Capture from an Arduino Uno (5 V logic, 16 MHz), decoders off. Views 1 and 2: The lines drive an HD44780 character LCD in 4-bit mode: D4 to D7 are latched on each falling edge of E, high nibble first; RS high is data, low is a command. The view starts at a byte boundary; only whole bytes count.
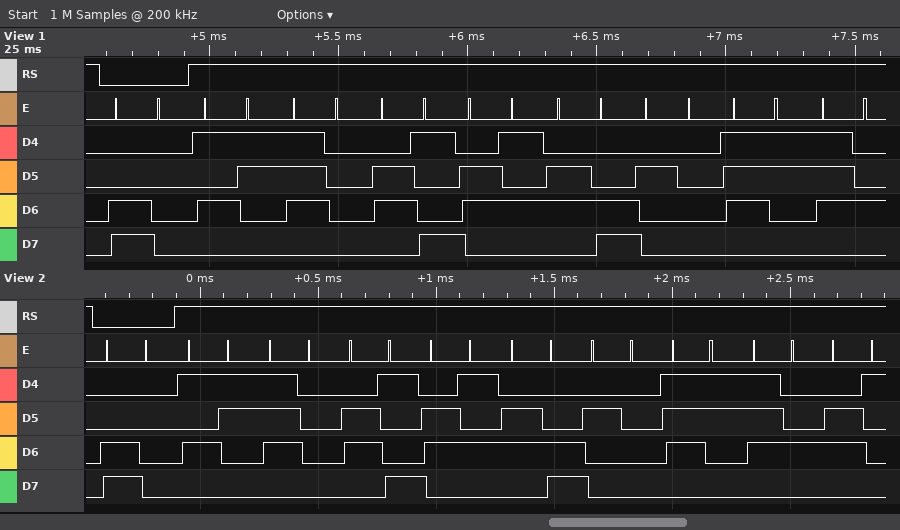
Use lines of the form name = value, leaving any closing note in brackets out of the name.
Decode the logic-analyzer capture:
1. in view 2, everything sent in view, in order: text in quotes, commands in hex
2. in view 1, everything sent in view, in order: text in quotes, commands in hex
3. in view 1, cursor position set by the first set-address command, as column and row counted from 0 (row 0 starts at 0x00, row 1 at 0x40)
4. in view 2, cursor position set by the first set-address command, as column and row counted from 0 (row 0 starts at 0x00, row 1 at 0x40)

in view 2, everything sent in view, in order: text in quotes, commands in hex = 0xC0 "Spiel sta"
in view 1, everything sent in view, in order: text in quotes, commands in hex = 0xC0 "Spiel st"
in view 1, cursor position set by the first set-address command, as column and row counted from 0 = column 0, row 1
in view 2, cursor position set by the first set-address command, as column and row counted from 0 = column 0, row 1
